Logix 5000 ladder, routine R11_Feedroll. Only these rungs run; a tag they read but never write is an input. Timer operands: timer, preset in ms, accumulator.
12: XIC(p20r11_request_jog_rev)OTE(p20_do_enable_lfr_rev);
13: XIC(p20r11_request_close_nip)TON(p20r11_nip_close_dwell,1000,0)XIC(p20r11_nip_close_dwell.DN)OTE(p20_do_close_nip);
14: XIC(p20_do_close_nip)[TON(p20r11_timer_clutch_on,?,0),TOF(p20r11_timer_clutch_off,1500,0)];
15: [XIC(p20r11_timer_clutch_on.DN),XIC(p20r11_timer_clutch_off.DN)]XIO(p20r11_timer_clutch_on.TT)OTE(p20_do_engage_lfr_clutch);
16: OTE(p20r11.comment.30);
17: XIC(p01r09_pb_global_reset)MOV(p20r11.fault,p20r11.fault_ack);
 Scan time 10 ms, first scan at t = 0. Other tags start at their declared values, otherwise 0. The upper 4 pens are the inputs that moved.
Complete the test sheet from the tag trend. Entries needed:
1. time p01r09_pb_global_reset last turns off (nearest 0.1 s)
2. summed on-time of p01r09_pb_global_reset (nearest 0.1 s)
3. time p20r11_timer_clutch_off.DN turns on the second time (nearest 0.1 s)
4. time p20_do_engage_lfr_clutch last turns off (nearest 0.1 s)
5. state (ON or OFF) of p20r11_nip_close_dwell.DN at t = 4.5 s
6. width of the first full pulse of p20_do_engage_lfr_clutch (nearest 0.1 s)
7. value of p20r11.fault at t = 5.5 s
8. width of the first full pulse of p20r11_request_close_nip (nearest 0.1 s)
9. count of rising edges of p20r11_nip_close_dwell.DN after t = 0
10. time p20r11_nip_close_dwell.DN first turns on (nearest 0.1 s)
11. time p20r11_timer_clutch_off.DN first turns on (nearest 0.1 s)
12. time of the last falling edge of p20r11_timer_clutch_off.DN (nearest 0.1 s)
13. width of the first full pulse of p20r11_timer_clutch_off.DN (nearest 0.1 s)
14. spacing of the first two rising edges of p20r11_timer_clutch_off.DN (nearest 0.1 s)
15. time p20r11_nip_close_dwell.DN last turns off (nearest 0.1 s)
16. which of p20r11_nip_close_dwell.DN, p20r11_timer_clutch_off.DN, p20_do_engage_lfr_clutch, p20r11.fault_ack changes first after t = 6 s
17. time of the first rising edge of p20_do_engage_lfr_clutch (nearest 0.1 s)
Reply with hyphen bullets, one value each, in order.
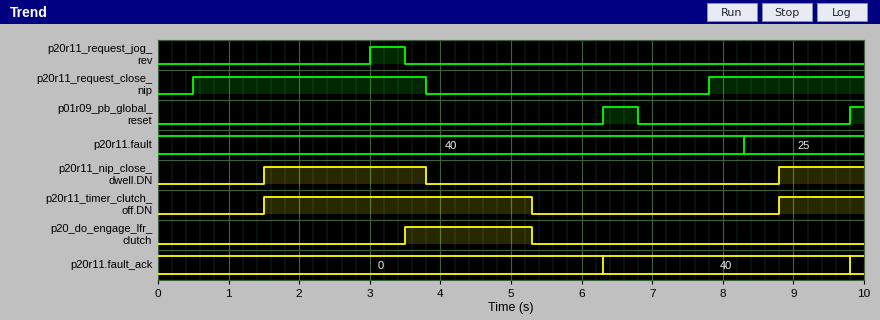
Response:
- 6.8 s
- 0.7 s
- 8.8 s
- 5.3 s
- OFF
- 1.8 s
- 40
- 3.3 s
- 2
- 1.5 s
- 1.5 s
- 5.3 s
- 3.8 s
- 7.3 s
- 3.8 s
- p20r11.fault_ack
- 3.5 s
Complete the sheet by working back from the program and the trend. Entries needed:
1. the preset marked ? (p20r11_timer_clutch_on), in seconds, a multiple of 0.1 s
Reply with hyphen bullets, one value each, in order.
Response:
- 2.0 s
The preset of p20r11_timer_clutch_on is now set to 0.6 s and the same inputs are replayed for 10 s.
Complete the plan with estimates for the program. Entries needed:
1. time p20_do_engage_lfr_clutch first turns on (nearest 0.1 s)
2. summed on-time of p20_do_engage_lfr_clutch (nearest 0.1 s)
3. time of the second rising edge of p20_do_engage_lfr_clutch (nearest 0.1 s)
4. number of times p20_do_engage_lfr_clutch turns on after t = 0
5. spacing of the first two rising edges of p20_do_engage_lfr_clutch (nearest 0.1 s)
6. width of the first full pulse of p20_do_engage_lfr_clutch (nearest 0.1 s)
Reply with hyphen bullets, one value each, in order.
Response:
- 2.1 s
- 3.8 s
- 9.4 s
- 2
- 7.3 s
- 3.2 s
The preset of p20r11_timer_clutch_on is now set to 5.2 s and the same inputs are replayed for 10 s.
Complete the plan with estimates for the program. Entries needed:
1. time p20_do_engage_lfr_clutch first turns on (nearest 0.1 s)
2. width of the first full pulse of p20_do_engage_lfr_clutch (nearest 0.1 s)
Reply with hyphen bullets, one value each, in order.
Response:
- 3.8 s
- 1.5 s
